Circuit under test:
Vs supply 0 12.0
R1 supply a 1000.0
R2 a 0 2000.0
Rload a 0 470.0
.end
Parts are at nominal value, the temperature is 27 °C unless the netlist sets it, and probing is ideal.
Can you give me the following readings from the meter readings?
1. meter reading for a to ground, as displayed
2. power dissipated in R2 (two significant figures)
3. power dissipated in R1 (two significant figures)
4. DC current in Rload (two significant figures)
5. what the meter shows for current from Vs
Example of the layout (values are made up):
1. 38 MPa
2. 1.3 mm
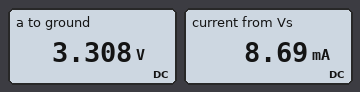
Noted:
1. 3.308 V
2. 5.5 mW
3. 76 mW
4. 7.0 mA
5. 8.69 mA
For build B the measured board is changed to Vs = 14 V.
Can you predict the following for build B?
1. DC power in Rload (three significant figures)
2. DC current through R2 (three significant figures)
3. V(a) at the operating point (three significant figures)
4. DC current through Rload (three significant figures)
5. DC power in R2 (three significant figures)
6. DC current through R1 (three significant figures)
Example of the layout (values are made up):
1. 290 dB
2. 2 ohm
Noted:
1. 31.7 mW
2. 1.93 mA
3. 3.86 V
4. 8.21 mA
5. 7.45 mW
6. 10.1 mA
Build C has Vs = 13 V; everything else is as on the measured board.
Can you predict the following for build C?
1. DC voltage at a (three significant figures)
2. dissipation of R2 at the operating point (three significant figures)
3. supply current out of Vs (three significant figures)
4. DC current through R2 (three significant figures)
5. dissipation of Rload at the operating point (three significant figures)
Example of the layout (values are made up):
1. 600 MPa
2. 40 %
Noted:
1. 3.58 V
2. 6.42 mW
3. 9.42 mA
4. 1.79 mA
5. 27.3 mW
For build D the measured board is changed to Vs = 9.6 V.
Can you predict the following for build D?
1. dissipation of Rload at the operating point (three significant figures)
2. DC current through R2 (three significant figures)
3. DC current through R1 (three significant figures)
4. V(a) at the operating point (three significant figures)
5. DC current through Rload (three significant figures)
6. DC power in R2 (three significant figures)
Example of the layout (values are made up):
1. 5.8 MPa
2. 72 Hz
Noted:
1. 14.9 mW
2. 1.32 mA
3. 6.95 mA
4. 2.65 V
5. 5.63 mA
6. 3.50 mW
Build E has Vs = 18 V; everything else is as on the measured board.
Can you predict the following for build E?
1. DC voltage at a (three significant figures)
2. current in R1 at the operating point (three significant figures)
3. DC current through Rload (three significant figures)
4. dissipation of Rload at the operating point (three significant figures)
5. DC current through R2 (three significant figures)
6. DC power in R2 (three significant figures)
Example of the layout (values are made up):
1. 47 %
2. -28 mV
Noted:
1. 4.96 V
2. 13.0 mA
3. 10.6 mA
4. 52.4 mW
5. 2.48 mA
6. 12.3 mW
